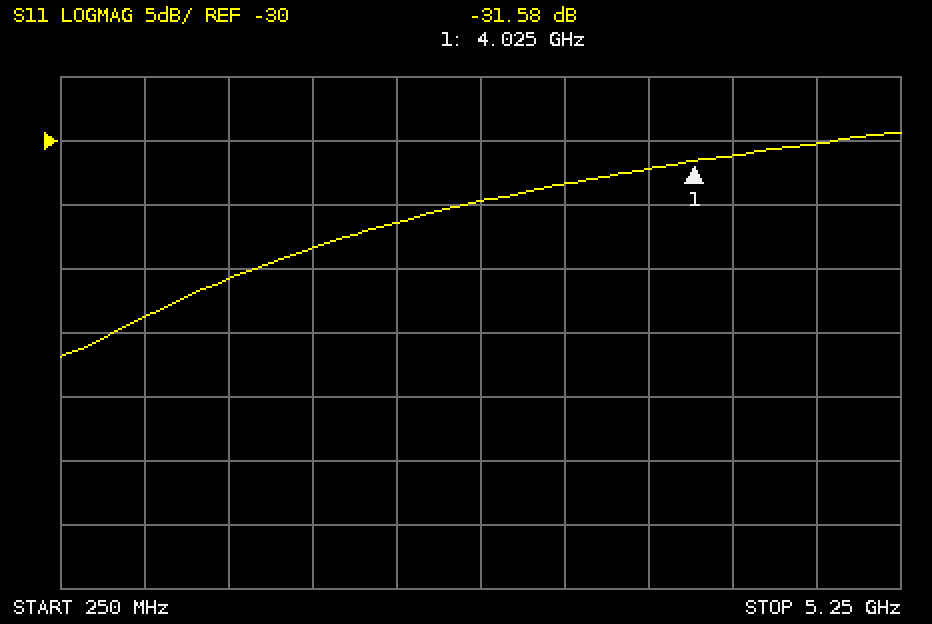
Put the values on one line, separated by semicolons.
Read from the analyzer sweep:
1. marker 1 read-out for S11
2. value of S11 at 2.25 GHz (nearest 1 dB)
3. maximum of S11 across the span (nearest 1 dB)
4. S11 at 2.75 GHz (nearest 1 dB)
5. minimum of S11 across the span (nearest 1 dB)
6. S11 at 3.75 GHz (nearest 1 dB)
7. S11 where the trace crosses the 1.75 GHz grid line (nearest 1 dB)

-31.58 dB; -36 dB; -29 dB; -35 dB; -47 dB; -32 dB; -38 dB
